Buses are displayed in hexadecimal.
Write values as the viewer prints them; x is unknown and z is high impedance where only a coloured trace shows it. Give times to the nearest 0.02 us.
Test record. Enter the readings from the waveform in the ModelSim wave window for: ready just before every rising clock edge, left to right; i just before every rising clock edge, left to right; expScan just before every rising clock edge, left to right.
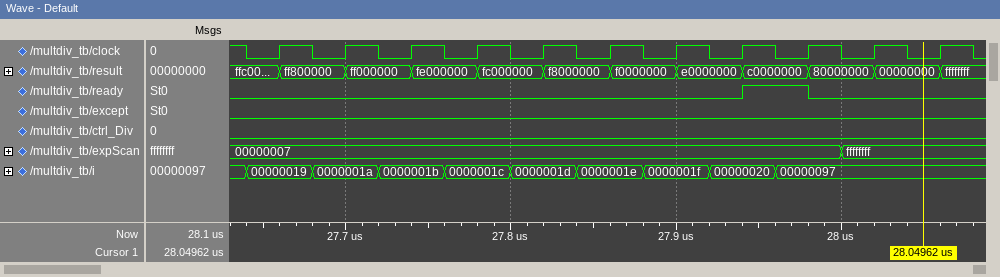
0 0 0 0 0 0 0 0 1 0 0
00000019, 0000001a, 0000001b, 0000001c, 0000001d, 0000001e, 0000001f, 00000020, 00000097, 00000097, 00000097
00000007, 00000007, 00000007, 00000007, 00000007, 00000007, 00000007, 00000007, 00000007, ffffffff, ffffffff
